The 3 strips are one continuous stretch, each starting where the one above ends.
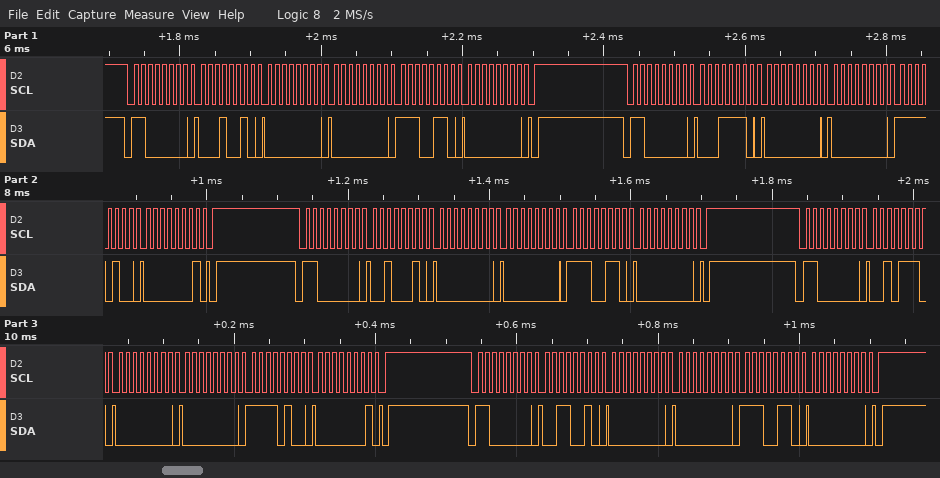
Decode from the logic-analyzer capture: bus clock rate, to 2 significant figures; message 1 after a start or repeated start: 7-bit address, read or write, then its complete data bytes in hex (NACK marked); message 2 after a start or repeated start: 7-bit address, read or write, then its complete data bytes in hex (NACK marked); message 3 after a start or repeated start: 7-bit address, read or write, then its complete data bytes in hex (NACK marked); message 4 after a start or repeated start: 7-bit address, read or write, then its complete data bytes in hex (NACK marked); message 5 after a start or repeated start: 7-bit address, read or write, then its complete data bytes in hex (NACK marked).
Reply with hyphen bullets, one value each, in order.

- 100 kHz
- 0x60 write: 12 00 00 E6 00
- 0x60 write: 1E 00 00 F4 01
- 0x60 write: 22 00 00 E6 00
- 0x60 write: 2E 00 00 F4 01
- 0x60 write: 32 00 00 E6 00
